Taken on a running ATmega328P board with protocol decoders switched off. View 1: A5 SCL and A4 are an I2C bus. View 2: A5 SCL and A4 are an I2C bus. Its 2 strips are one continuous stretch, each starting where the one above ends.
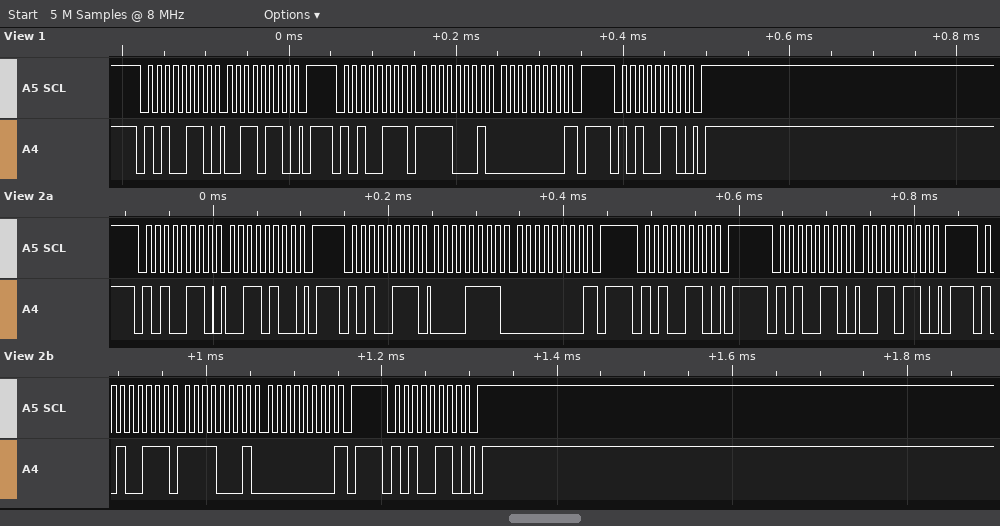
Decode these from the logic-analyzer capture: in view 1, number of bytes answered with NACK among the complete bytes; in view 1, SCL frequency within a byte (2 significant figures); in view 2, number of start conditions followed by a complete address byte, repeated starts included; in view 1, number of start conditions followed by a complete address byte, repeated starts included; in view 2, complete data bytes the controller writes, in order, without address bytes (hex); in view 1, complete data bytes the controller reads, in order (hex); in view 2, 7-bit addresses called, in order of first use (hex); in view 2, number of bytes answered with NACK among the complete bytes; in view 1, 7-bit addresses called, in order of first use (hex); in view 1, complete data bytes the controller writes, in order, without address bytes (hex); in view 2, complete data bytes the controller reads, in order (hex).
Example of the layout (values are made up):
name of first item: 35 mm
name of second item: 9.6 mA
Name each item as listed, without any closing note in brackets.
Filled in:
in view 1, number of bytes answered with NACK among the complete bytes: 1
in view 1, SCL frequency within a byte: 100 kHz
in view 2, number of start conditions followed by a complete address byte, repeated starts included: 6
in view 1, number of start conditions followed by a complete address byte, repeated starts included: 3
in view 2, complete data bytes the controller writes, in order, without address bytes: 34 36
in view 1, complete data bytes the controller reads, in order: F1 00
in view 2, 7-bit addresses called, in order of first use: 0x53
in view 2, number of bytes answered with NACK among the complete bytes: 2
in view 1, 7-bit addresses called, in order of first use: 0x53
in view 1, complete data bytes the controller writes, in order, without address bytes: 36
in view 2, complete data bytes the controller reads, in order: 0F 00 F1 00
